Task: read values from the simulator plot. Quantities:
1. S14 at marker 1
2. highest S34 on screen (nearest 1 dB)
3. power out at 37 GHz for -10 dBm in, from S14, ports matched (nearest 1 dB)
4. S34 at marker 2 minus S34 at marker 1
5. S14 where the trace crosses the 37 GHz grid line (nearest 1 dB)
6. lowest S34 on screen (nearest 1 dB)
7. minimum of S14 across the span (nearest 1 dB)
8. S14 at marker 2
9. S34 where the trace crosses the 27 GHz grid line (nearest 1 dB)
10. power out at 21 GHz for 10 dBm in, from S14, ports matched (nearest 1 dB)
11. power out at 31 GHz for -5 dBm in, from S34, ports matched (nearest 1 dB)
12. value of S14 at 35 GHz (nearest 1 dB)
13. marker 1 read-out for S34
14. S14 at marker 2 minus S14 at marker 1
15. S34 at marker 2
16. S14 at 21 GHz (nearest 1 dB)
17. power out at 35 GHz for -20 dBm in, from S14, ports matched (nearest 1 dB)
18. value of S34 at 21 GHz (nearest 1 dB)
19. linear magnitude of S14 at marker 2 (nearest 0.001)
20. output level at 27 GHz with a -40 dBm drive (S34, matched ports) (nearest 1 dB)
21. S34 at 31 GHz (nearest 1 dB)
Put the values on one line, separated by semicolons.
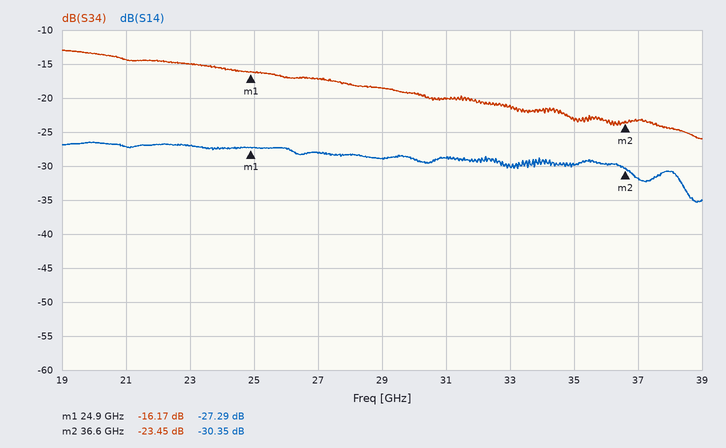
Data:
-27.29 dB; -13 dB; -42 dBm; -7.28 dB; -32 dB; -26 dB; -35 dB; -30.35 dB; -17 dB; -17 dBm; -25 dBm; -30 dB; -16.17 dB; -3.06 dB; -23.45 dB; -27 dB; -50 dBm; -14 dB; 0.030; -57 dBm; -20 dB
